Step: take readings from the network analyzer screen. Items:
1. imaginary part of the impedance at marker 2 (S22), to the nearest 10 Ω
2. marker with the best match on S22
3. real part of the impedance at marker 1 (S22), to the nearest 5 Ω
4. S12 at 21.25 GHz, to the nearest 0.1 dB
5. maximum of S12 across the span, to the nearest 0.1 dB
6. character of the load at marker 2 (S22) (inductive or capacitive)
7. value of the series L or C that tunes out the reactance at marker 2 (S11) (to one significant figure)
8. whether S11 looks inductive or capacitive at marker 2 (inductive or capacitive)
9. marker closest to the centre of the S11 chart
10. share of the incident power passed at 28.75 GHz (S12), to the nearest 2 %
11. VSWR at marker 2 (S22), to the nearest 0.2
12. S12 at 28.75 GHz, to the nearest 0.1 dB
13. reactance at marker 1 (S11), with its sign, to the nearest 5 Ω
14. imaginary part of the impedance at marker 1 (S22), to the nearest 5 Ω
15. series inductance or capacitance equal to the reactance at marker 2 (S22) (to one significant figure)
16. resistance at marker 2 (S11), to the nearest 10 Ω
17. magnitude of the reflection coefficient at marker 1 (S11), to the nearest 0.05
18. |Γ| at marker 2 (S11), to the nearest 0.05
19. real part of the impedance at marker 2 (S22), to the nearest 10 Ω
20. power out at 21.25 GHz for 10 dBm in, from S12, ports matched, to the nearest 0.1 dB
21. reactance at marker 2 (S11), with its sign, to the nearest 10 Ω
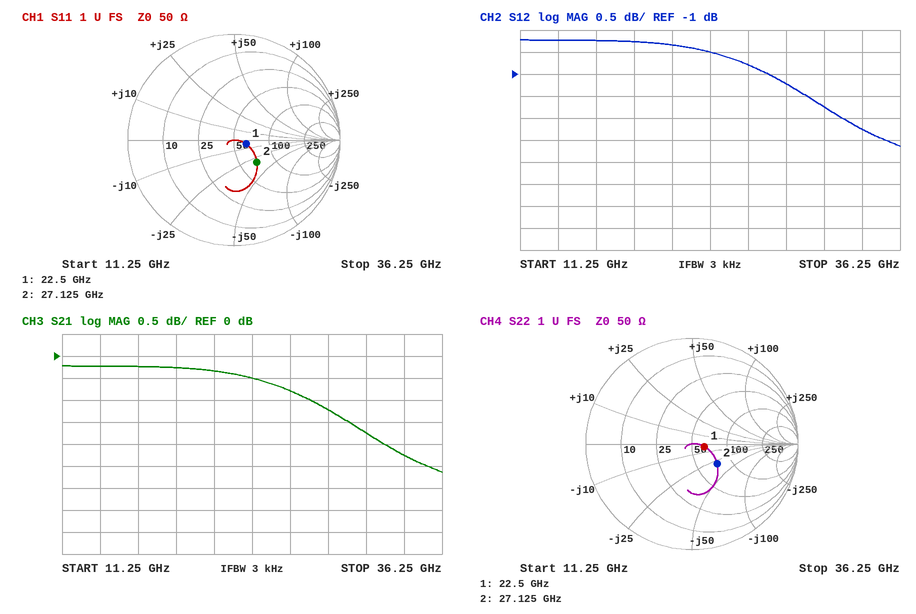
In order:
-30 Ω
marker 1
65 Ω
-0.3 dB
-0.2 dB
capacitive
200 pH
capacitive
marker 1
76 %
1.8
-1.2 dB
-5 Ω
-5 Ω
200 fF
70 Ω
0.10
0.30
70 Ω
9.7 dBm
-30 Ω
